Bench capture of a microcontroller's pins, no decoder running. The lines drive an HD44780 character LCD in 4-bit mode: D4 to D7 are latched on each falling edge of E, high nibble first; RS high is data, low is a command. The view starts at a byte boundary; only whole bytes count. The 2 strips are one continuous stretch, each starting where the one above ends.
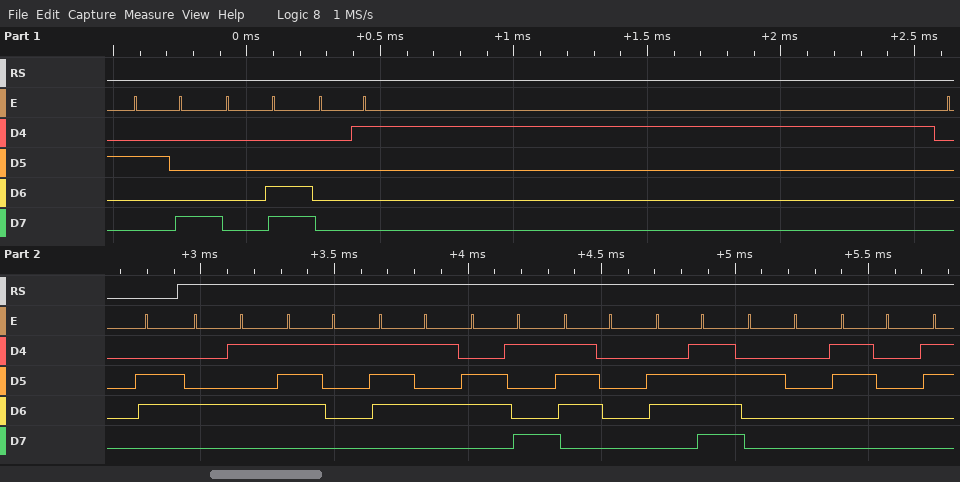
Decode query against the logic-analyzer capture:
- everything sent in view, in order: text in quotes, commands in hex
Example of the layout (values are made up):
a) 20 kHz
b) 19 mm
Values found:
a) 0x28 0x0C 0x01 0x06 "Equipo 0"
